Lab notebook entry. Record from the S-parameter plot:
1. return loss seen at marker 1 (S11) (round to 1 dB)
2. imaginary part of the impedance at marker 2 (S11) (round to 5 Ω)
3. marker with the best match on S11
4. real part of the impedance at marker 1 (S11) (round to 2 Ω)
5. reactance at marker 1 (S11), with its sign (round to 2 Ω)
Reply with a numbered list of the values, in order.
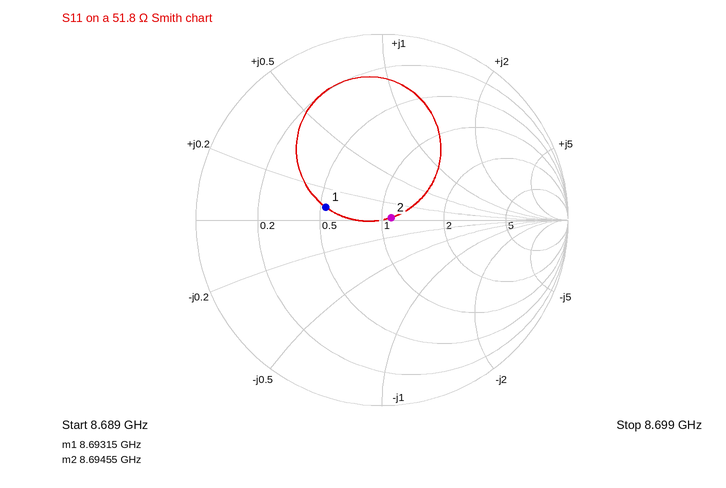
1. 10 dB
2. 0 Ω
3. marker 2
4. 28 Ω
5. +4 Ω
